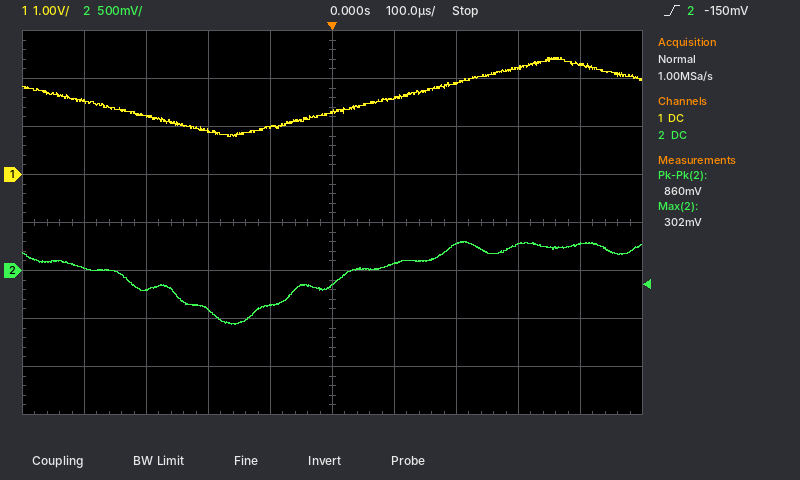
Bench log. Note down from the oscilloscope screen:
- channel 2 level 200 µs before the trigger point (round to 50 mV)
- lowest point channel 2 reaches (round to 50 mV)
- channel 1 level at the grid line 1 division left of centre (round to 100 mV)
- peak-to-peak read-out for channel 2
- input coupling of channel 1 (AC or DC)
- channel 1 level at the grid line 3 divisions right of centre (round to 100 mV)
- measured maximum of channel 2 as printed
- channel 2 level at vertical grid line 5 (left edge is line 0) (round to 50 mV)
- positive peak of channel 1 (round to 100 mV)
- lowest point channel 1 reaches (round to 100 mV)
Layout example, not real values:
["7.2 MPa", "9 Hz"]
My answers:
["-400 mV", "-550 mV", "1.0 V", "860 mV", "DC", "2.2 V", "302 mV", "-150 mV", "2.4 V", "800 mV"]
